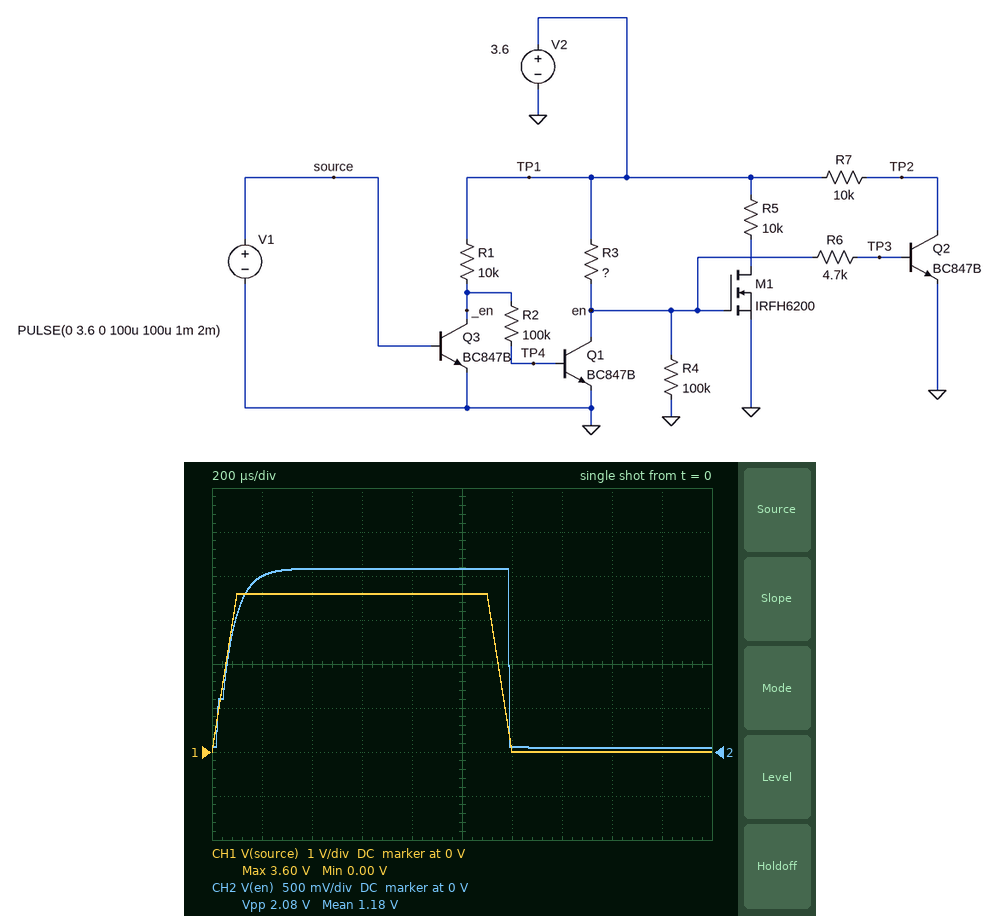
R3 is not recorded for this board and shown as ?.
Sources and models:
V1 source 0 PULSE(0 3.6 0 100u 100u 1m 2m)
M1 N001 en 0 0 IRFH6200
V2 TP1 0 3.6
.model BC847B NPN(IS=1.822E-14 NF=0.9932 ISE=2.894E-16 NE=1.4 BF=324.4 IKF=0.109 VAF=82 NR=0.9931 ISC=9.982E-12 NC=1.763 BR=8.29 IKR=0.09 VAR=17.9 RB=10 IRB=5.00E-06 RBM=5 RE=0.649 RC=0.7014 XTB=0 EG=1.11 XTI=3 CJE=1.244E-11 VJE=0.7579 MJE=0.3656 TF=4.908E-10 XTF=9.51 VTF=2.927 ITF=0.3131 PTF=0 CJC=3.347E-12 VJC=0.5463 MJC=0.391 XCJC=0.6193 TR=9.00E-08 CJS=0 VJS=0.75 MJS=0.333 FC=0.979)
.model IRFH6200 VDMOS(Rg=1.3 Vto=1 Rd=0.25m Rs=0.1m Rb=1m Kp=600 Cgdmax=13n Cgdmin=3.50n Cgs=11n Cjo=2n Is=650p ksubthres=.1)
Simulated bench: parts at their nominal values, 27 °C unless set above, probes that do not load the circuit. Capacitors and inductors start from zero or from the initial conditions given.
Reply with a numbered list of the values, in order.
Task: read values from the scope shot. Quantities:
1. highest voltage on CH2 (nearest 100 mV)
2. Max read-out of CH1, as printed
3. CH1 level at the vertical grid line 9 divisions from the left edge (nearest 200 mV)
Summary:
1. 2.1 V
2. 3.60 V
3. 0 V
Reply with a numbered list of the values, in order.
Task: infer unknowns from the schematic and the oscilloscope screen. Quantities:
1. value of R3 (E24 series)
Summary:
1. 4.7 kΩ
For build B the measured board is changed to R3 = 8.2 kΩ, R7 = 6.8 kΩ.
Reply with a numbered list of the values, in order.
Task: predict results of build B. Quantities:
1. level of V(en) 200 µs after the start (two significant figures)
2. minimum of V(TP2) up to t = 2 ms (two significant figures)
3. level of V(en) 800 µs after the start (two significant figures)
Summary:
1. 1.5 V
2. 11 mV
3. 1.7 V
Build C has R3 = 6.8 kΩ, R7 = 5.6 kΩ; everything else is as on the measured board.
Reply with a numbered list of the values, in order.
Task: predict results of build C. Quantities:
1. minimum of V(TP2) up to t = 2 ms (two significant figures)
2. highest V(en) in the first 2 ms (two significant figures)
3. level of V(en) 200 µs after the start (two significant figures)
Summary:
1. 12 mV
2. 1.8 V
3. 1.7 V
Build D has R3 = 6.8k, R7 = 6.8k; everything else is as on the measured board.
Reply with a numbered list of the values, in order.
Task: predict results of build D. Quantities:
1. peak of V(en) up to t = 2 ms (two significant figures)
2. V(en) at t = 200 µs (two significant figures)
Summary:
1. 1.8 V
2. 1.7 V
